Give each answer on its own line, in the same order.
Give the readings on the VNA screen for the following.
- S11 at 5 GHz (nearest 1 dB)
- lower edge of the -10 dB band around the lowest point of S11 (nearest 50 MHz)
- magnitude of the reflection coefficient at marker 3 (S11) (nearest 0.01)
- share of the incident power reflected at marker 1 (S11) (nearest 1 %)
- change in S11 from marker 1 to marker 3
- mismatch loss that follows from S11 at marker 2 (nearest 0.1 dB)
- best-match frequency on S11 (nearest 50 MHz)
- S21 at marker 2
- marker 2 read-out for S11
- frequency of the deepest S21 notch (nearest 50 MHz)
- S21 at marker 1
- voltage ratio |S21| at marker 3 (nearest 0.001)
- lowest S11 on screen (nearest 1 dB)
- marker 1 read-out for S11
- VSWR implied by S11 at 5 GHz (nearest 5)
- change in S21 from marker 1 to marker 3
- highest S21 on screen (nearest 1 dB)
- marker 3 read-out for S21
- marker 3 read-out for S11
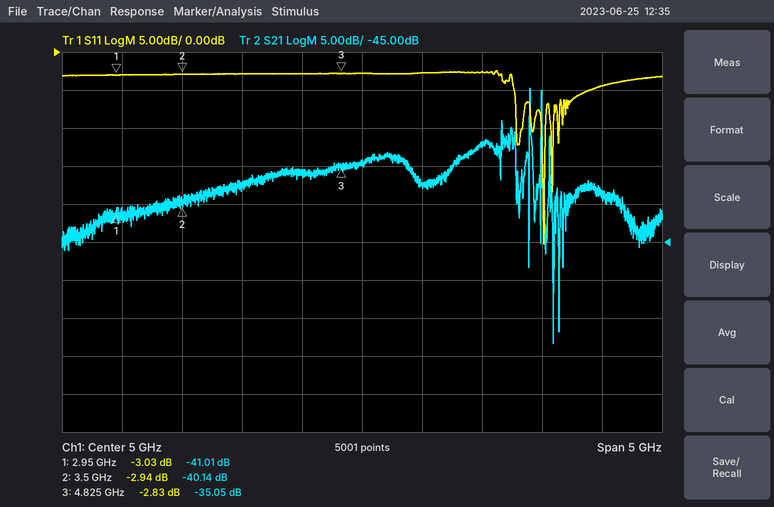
-3 dB
6.50 GHz
0.72
50 %
0.20 dB
3.1 dB
6.50 GHz
-40.14 dB
-2.94 dB
6.60 GHz
-41.01 dB
0.018
-25 dB
-3.03 dB
5
5.96 dB
-25 dB
-35.05 dB
-2.83 dB
